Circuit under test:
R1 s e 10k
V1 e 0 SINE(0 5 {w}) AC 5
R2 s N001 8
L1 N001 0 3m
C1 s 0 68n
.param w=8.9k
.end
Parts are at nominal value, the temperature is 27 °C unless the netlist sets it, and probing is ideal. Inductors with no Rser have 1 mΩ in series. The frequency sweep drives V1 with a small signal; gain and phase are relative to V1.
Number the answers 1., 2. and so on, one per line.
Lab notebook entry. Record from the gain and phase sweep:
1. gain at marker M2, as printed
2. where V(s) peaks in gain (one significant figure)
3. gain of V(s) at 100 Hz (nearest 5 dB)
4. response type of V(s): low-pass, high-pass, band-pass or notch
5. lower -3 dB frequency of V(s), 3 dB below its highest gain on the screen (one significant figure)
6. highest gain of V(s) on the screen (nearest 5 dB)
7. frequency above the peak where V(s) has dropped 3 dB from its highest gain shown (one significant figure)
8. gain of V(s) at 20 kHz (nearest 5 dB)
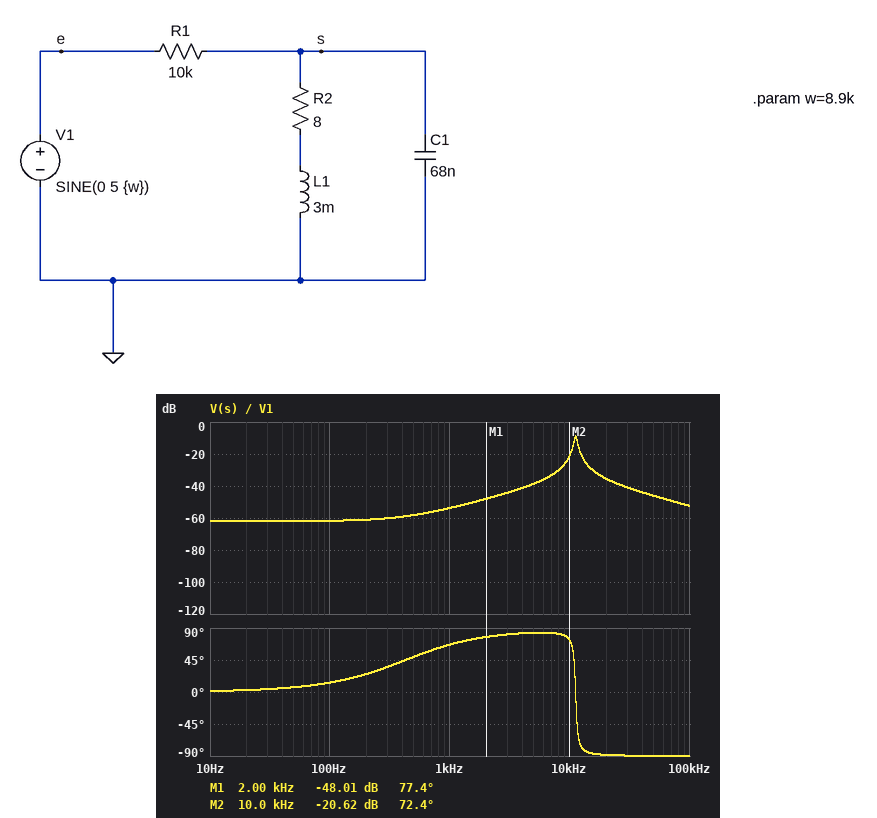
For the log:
1. -20.62 dB
2. 10 kHz
3. -60 dB
4. band-pass
5. 10 kHz
6. -10 dB
7. 10 kHz
8. -35 dB
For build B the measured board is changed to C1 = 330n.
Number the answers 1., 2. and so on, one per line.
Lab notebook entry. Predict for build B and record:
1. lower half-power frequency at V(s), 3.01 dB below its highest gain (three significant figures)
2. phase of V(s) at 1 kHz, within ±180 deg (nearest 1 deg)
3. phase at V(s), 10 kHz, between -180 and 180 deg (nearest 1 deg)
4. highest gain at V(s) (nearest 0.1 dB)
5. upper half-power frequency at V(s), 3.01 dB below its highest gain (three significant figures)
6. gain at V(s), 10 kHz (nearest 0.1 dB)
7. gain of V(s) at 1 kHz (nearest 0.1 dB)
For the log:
1. 4.83 kHz
2. 66 deg
3. -89 deg
4. -19.8 dB
5. 5.30 kHz
6. -43.8 dB
7. -53.4 dB
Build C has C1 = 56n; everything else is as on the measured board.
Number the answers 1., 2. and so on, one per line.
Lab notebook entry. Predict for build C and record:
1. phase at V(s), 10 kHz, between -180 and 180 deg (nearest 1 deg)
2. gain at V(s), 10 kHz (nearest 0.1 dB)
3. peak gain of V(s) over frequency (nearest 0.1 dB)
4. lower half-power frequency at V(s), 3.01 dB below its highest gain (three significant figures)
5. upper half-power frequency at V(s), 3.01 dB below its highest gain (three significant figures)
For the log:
1. 80 deg
2. -25.1 dB
3. -7.9 dB
4. 11.9 kHz
5. 12.6 kHz
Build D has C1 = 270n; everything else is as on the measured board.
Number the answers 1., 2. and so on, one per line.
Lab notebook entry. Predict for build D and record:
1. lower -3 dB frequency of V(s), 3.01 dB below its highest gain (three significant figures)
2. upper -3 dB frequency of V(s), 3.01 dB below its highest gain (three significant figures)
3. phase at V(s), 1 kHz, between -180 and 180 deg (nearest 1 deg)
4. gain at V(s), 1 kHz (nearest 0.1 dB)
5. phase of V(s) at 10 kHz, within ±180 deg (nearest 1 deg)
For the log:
1. 5.36 kHz
2. 5.84 kHz
3. 66 deg
4. -53.5 dB
5. -88 deg
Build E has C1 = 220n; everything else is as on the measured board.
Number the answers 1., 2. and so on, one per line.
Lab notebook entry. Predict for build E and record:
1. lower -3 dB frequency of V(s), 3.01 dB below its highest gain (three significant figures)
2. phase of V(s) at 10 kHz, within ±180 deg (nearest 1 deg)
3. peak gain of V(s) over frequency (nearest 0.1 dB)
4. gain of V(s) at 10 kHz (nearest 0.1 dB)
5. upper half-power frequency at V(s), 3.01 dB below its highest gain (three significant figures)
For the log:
1. 5.95 kHz
2. -88 deg
3. -16.7 dB
4. -38.6 dB
5. 6.45 kHz
